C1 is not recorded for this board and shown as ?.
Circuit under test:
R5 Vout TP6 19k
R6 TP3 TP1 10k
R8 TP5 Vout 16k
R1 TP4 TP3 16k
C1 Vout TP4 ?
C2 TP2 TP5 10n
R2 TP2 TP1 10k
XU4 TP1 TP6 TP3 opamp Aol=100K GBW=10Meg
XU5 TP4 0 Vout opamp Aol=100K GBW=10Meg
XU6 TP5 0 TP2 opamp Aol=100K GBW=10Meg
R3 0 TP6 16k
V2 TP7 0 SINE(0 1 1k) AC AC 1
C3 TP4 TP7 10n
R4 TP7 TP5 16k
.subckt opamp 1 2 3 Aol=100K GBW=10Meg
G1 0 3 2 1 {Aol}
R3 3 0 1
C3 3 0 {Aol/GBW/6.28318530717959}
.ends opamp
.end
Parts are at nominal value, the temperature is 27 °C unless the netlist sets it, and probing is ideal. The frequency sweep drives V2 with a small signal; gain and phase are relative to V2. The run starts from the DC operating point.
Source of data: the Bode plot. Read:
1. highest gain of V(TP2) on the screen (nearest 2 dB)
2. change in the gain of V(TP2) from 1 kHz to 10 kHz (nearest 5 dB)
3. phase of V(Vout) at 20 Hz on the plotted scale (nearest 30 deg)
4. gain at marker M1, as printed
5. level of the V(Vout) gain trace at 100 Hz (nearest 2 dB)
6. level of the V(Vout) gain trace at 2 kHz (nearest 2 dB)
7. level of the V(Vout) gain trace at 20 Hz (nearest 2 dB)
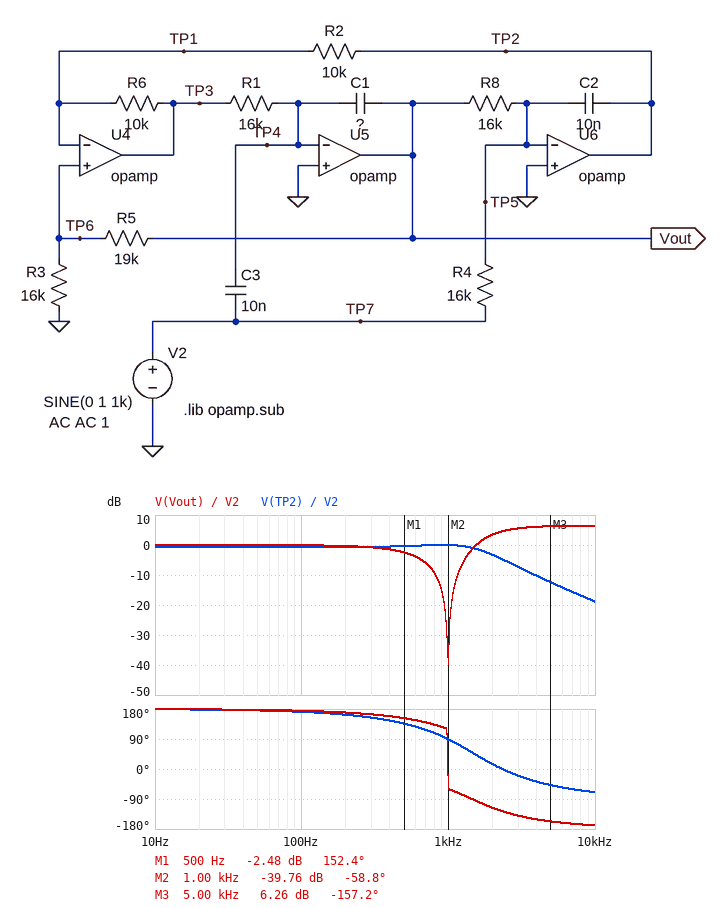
0 dB
-20 dB
180 deg
-2.48 dB
0 dB
4 dB
0 dB
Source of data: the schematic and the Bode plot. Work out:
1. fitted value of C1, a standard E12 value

4.7 nF
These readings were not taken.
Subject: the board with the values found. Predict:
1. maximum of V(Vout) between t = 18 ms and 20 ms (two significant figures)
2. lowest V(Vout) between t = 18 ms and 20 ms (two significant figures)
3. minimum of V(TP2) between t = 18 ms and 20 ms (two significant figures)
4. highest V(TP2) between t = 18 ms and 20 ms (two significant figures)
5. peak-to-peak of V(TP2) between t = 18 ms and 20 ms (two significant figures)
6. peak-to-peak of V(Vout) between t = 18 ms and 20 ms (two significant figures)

10 mV
-10 mV
-1.0 V
1.0 V
2.0 V
21 mV
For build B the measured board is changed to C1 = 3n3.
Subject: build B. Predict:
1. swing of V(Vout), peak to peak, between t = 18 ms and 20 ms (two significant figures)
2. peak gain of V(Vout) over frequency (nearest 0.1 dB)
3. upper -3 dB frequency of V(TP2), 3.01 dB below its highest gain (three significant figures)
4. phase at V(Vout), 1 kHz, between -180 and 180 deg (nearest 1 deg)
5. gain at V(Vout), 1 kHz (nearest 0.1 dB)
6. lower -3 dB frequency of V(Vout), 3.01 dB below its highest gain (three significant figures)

19 mV
9.6 dB
2.71 kHz
-53 deg
-40.4 dB
2.57 kHz
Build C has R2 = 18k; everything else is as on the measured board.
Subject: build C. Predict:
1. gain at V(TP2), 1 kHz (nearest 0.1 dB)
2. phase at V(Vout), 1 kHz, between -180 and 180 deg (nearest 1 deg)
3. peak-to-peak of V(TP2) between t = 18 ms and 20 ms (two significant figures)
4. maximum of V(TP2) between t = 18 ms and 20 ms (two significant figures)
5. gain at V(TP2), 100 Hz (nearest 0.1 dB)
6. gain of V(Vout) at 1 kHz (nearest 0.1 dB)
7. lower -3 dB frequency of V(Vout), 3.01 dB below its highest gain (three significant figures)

1.8 dB
-84 deg
2.5 V
1.2 V
2.2 dB
-4.0 dB
1.56 kHz
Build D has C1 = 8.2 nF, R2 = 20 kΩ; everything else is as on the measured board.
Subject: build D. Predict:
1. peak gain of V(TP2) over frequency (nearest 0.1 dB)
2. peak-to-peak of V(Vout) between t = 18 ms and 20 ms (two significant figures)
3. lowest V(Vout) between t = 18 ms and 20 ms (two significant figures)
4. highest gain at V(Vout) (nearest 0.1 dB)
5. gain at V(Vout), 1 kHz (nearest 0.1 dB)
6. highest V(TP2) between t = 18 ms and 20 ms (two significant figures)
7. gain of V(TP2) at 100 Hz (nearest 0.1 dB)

3.7 dB
1.3 V
-670 mV
1.7 dB
-3.5 dB
930 mV
2.8 dB
